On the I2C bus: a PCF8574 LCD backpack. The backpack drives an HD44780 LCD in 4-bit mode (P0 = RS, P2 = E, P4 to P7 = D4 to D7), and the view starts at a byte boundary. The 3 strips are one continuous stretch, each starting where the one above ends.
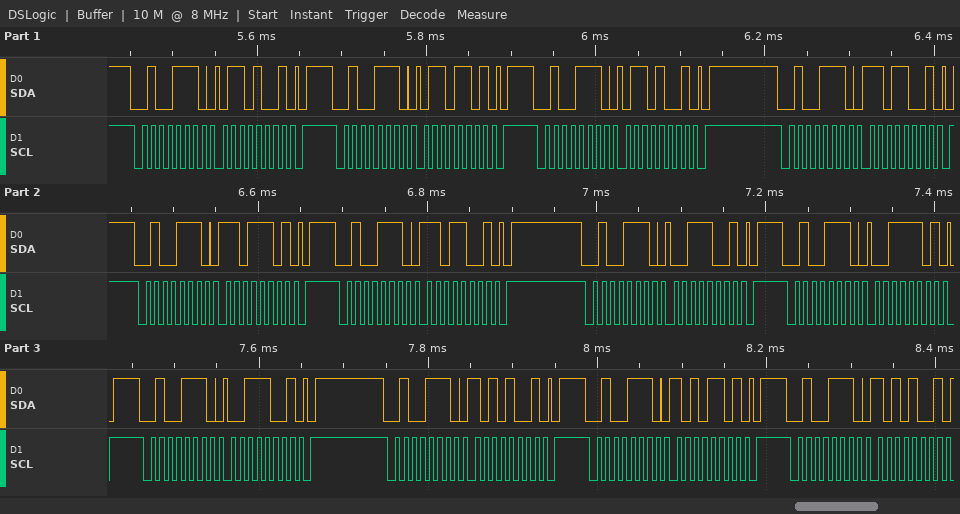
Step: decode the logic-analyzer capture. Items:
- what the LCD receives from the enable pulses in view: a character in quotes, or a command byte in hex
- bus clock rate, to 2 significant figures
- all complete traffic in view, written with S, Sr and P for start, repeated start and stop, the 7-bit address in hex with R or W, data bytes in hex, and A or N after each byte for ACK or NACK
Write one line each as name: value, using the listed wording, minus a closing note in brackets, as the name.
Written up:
what the LCD receives from the enable pulses in view: a character in quotes, or a command byte in hex: 'm' ':'
bus clock rate, to 2 significant figures: 100 kHz
all complete traffic in view, written with S, Sr and P for start, repeated start and stop, the 7-bit address in hex with R or W, data bytes in hex, and A or N after each byte for ACK or NACK: S 27W A 69 A P S 27W A 6D A P S 27W A 69 A P S 27W A D9 A P S 27W A DD A P S 27W A D9 A P S 27W A 39 A P S 27W A 3D A P S 27W A 39 A P S 27W A A9 A P S 27W A AD A P S 27W A A9 A
